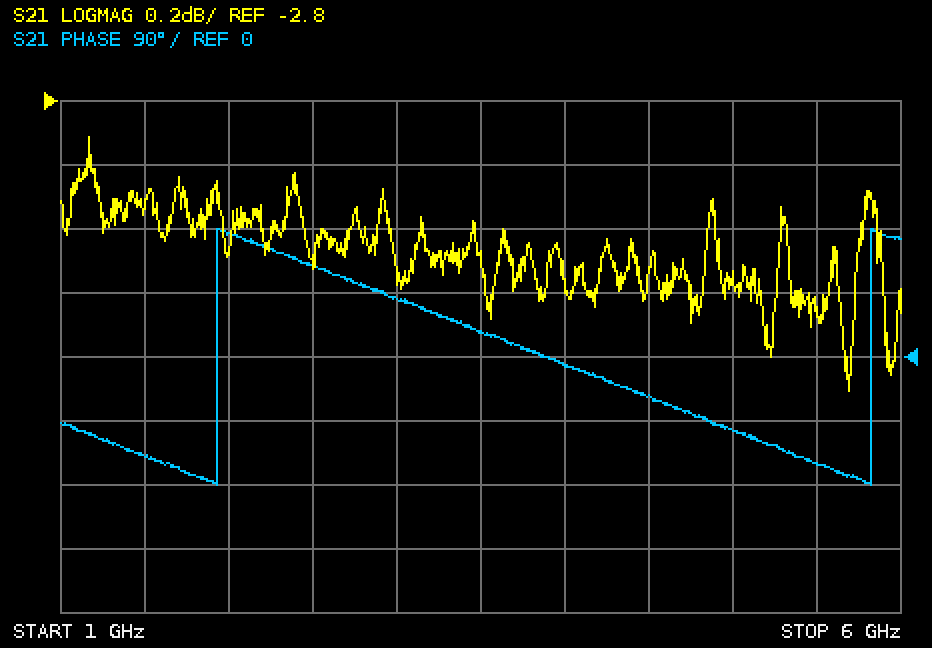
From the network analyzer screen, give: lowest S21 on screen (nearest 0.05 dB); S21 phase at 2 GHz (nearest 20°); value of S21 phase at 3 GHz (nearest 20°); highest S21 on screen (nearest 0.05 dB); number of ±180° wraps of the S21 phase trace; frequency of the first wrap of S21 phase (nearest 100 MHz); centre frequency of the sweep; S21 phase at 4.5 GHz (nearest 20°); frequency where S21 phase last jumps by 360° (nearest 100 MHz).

-3.70 dB
180°
80°
-2.90 dB
2
1.9 GHz
3.5 GHz
-60°
5.8 GHz
